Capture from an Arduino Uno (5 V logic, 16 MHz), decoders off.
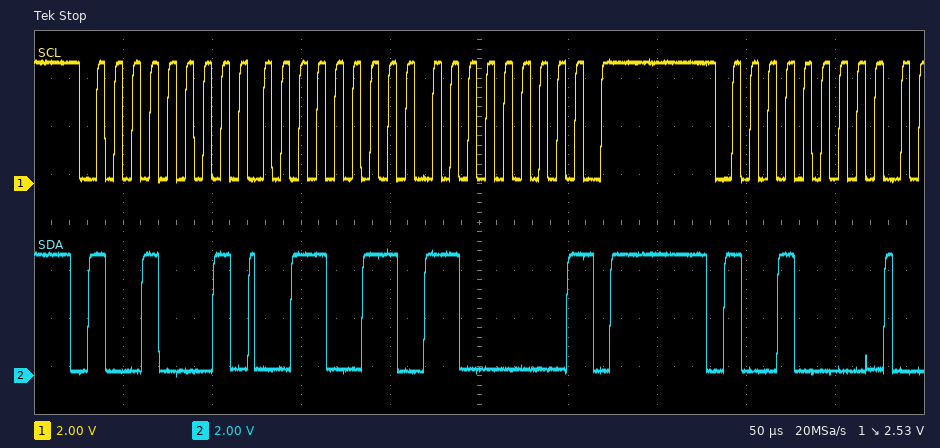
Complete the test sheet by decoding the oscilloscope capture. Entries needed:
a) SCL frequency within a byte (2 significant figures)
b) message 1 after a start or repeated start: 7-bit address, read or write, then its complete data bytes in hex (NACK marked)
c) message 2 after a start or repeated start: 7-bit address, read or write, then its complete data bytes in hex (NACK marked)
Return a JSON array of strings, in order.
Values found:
["100 kHz", "0x48 read: 33 C0 NACK", "0x48 write"]
